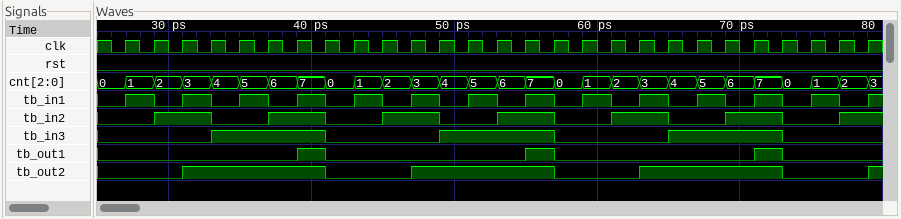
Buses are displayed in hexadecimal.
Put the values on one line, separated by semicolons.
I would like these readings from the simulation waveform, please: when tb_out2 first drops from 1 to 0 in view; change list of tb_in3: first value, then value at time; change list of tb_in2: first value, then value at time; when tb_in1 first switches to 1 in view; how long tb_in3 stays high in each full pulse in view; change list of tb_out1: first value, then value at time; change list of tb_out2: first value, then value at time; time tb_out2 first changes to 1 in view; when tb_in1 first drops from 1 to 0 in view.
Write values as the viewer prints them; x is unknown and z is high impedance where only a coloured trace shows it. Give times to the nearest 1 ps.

41 ps; 0, 1 at 33 ps, 0 at 41 ps, 1 at 49 ps, 0 at 57 ps, 1 at 65 ps, 0 at 73 ps; 0, 1 at 29 ps, 0 at 33 ps, 1 at 37 ps, 0 at 41 ps, 1 at 45 ps, 0 at 49 ps, 1 at 53 ps, 0 at 57 ps, 1 at 61 ps, 0 at 65 ps, 1 at 69 ps, 0 at 73 ps, 1 at 77 ps; 27 ps; 8 ps, 8 ps, 8 ps; 0, 1 at 39 ps, 0 at 41 ps, 1 at 55 ps, 0 at 57 ps, 1 at 71 ps, 0 at 73 ps; 0, 1 at 31 ps, 0 at 41 ps, 1 at 47 ps, 0 at 57 ps, 1 at 63 ps, 0 at 73 ps, 1 at 79 ps; 31 ps; 29 ps
